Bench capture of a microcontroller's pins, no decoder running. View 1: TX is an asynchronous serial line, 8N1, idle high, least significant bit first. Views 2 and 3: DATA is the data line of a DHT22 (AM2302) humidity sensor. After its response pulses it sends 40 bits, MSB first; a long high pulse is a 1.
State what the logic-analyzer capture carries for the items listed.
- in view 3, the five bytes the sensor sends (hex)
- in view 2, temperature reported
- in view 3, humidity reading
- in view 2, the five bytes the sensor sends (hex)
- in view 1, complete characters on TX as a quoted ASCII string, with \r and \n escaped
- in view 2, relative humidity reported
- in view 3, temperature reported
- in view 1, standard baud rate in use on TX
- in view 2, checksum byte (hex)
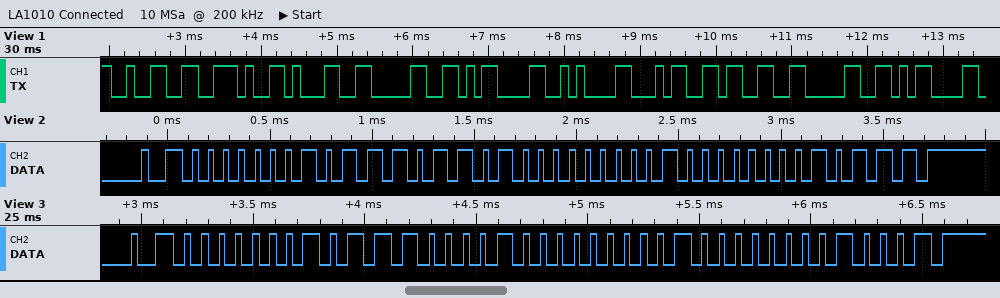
01 70 80 20 11
-3.2 °C
36.8 %
01 76 80 20 17
"2.10\r\n430\r"
37.4 %
-3.2 °C
9600 baud
0x17
